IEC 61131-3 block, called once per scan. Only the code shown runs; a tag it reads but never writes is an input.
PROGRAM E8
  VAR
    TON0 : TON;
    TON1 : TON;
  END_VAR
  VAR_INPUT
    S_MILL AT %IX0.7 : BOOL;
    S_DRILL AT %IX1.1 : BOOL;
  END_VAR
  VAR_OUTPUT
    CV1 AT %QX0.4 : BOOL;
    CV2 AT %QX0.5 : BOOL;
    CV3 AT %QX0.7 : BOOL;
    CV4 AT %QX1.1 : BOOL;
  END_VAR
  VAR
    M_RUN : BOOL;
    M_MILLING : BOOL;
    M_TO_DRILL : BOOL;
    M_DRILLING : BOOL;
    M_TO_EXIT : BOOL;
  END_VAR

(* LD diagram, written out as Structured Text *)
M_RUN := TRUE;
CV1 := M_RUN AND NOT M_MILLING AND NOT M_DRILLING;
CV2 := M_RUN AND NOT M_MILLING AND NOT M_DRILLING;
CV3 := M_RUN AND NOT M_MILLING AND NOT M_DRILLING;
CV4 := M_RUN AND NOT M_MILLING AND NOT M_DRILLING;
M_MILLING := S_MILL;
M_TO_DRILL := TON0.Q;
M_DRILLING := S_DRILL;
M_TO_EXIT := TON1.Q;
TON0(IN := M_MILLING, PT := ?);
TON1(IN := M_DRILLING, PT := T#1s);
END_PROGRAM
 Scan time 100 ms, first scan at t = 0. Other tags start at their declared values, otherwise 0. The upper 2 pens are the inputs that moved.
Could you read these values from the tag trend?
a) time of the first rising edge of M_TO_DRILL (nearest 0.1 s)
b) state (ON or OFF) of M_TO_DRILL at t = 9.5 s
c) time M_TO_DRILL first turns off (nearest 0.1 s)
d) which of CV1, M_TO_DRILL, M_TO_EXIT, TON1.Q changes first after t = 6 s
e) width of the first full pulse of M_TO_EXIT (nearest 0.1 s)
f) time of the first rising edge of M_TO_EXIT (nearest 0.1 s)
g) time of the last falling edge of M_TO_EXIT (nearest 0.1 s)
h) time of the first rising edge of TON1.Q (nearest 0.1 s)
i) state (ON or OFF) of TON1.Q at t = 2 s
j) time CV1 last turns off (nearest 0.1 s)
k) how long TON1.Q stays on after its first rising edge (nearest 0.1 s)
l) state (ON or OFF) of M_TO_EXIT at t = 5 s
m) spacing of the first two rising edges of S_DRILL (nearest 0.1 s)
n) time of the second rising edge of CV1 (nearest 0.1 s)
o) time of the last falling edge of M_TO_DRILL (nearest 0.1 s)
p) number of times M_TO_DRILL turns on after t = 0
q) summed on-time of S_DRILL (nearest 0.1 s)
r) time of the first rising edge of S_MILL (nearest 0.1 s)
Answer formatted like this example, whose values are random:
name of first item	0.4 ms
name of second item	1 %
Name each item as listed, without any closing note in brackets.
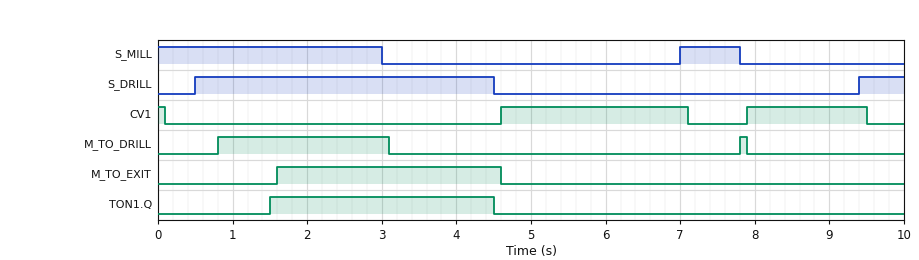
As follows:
time of the first rising edge of M_TO_DRILL	0.8 s
state (ON or OFF) of M_TO_DRILL at t = 9.5 s	OFF
time M_TO_DRILL first turns off	3.1 s
which of CV1, M_TO_DRILL, M_TO_EXIT, TON1.Q changes first after t = 6 s	CV1
width of the first full pulse of M_TO_EXIT	3.0 s
time of the first rising edge of M_TO_EXIT	1.6 s
time of the last falling edge of M_TO_EXIT	4.6 s
time of the first rising edge of TON1.Q	1.5 s
state (ON or OFF) of TON1.Q at t = 2 s	ON
time CV1 last turns off	9.5 s
how long TON1.Q stays on after its first rising edge	3.0 s
state (ON or OFF) of M_TO_EXIT at t = 5 s	OFF
spacing of the first two rising edges of S_DRILL	8.9 s
time of the second rising edge of CV1	7.9 s
time of the last falling edge of M_TO_DRILL	7.9 s
number of times M_TO_DRILL turns on after t = 0	2
summed on-time of S_DRILL	4.6 s
time of the first rising edge of S_MILL	7.0 s
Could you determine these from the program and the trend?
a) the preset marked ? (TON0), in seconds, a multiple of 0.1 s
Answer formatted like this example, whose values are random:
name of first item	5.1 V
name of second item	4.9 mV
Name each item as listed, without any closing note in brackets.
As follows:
the preset marked ? (TON0), in seconds, a multiple of 0.1 s	0.7 s
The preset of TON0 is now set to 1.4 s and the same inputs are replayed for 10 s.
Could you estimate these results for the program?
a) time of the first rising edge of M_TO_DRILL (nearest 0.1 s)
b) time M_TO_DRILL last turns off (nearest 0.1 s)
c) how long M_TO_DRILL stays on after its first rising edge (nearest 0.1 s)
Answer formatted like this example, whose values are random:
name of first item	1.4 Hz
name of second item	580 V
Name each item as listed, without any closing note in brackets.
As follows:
time of the first rising edge of M_TO_DRILL	1.5 s
time M_TO_DRILL last turns off	3.1 s
how long M_TO_DRILL stays on after its first rising edge	1.6 s
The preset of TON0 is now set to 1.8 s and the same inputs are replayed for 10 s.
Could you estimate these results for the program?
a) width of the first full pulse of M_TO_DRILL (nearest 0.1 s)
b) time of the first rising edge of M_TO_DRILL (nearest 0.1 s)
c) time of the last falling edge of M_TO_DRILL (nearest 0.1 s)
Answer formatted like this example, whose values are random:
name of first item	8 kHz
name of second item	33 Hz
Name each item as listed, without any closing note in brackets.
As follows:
width of the first full pulse of M_TO_DRILL	1.2 s
time of the first rising edge of M_TO_DRILL	1.9 s
time of the last falling edge of M_TO_DRILL	3.1 s
